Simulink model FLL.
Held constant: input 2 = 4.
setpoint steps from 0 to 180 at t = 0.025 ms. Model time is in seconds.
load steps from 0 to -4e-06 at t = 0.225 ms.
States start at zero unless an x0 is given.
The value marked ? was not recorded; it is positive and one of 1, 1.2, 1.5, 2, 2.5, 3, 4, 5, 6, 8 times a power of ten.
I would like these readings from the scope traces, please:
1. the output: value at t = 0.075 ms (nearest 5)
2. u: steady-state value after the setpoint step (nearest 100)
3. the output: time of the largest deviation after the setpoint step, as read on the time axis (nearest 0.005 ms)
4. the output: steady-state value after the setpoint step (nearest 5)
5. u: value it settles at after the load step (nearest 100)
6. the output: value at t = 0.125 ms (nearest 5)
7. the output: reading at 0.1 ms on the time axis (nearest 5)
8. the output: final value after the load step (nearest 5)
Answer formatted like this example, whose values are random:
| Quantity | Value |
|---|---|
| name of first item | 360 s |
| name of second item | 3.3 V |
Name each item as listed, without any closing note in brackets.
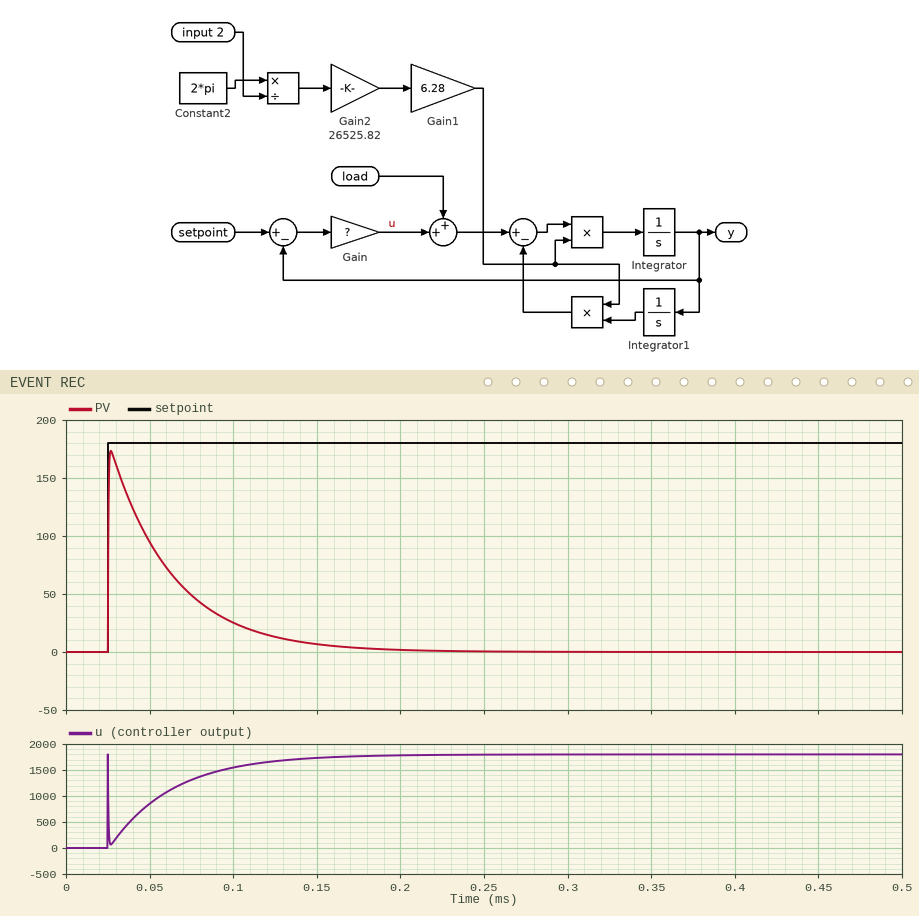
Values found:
| Quantity | Value |
|---|---|
| the output: value at t = 0.075 ms | 50 |
| u: steady-state value after the setpoint step | 1800 |
| the output: time of the largest deviation after the setpoint step, as read on the time axis | 0.025 ms |
| the output: steady-state value after the setpoint step | 0 |
| u: value it settles at after the load step | 1800 |
| the output: value at t = 0.125 ms | 15 |
| the output: reading at 0.1 ms on the time axis | 25 |
| the output: final value after the load step | 0 |
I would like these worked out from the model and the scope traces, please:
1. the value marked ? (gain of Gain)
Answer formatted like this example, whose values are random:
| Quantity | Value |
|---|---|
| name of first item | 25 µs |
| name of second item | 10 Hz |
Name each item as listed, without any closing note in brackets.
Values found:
| Quantity | Value |
|---|---|
| the value marked ? | 10 |
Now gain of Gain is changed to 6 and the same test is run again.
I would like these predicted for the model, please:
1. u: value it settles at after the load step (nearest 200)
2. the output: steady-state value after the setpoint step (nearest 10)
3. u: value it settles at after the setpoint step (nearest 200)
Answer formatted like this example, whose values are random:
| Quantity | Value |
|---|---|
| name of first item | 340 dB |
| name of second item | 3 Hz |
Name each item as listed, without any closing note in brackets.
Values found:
| Quantity | Value |
|---|---|
| u: value it settles at after the load step | 1000 |
| the output: steady-state value after the setpoint step | 0 |
| u: value it settles at after the setpoint step | 1000 |
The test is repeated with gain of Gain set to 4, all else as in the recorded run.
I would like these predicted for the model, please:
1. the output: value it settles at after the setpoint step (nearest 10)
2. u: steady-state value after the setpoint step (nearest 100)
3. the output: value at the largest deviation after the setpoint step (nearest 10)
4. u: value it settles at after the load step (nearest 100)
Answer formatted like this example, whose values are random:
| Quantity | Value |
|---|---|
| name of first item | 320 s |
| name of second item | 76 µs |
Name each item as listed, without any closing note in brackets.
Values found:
| Quantity | Value |
|---|---|
| the output: value it settles at after the setpoint step | 0 |
| u: steady-state value after the setpoint step | 700 |
| the output: value at the largest deviation after the setpoint step | 160 |
| u: value it settles at after the load step | 700 |
